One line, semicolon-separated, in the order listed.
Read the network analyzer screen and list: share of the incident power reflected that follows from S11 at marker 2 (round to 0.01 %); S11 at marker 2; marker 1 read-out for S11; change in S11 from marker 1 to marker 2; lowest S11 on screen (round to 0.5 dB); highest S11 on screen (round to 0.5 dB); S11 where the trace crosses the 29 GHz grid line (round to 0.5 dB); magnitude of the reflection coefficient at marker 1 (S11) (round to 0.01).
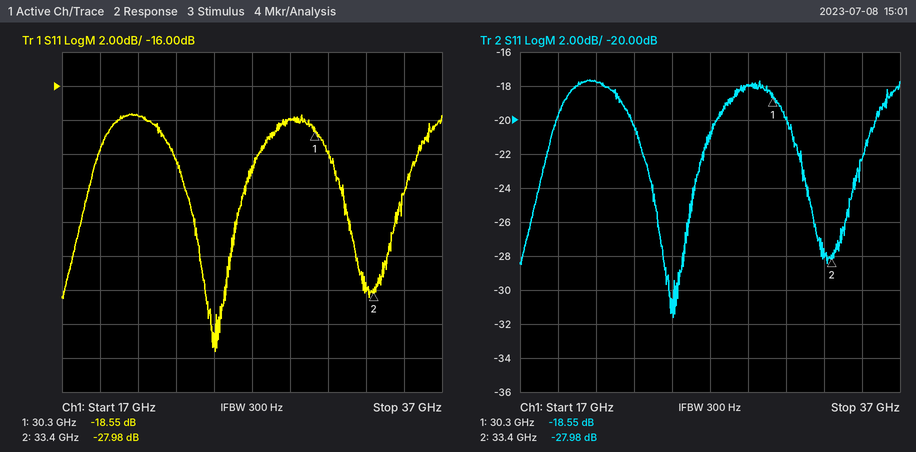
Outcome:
0.16 %; -27.98 dB; -18.55 dB; -9.43 dB; -31.5 dB; -17.5 dB; -18.0 dB; 0.12
